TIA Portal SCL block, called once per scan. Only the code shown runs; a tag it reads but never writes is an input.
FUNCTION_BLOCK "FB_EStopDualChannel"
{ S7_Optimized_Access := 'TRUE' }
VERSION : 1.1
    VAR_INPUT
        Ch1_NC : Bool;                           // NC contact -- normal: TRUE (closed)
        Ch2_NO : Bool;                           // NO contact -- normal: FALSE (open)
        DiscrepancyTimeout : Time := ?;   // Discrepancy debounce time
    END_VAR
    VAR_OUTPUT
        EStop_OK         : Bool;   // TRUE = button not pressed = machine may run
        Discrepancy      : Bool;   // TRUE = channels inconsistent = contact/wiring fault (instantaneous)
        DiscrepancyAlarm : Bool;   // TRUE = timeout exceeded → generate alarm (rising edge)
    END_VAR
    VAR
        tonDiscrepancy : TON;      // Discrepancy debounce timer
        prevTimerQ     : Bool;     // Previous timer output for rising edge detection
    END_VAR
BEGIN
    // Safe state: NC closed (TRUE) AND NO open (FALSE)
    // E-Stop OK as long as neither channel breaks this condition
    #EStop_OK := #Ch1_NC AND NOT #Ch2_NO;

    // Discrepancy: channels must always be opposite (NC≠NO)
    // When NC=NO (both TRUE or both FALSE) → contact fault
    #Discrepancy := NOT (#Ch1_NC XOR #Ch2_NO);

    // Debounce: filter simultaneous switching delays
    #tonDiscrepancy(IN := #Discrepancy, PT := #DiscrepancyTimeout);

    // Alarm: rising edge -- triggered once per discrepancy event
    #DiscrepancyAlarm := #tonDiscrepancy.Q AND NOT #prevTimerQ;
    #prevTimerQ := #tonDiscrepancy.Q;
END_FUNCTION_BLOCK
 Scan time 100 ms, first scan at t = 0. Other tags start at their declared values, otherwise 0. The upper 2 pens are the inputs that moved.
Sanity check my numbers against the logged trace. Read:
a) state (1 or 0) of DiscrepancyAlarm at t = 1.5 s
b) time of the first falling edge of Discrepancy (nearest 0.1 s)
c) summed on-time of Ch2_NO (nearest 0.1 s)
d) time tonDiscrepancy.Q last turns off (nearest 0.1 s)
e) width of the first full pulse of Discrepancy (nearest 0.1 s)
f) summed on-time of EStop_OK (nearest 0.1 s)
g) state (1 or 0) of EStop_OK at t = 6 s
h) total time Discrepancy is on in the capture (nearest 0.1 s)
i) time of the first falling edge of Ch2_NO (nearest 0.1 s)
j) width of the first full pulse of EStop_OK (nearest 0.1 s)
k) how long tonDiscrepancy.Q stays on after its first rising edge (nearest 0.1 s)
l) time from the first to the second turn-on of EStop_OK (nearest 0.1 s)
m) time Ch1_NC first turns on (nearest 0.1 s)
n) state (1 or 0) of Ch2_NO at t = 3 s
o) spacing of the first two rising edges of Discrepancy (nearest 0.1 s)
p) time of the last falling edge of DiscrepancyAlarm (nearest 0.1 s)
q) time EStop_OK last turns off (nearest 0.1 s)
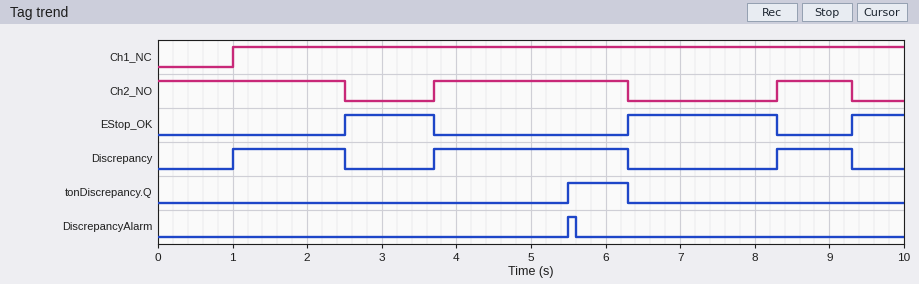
0
2.5 s
6.1 s
6.3 s
1.5 s
3.9 s
0
5.1 s
2.5 s
1.2 s
0.8 s
3.8 s
1.0 s
0
2.7 s
5.6 s
8.3 s
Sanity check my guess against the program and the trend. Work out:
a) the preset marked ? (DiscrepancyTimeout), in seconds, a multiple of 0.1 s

1.8 s
